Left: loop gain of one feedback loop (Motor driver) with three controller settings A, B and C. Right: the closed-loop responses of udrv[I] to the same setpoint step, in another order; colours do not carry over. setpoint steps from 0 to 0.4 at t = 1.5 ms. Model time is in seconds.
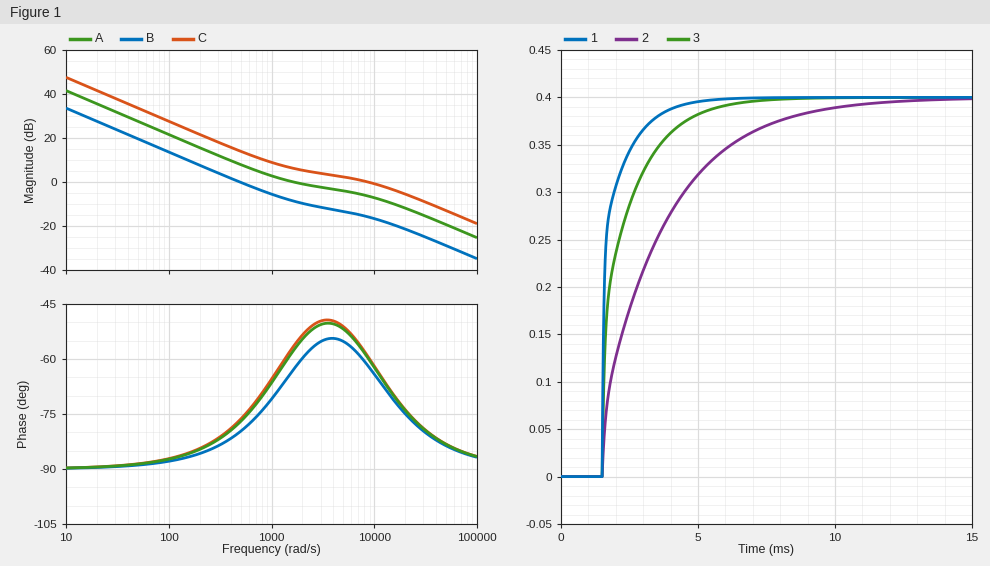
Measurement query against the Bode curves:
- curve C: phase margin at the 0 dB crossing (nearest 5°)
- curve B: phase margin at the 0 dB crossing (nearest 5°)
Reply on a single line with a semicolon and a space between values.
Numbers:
120°; 100°
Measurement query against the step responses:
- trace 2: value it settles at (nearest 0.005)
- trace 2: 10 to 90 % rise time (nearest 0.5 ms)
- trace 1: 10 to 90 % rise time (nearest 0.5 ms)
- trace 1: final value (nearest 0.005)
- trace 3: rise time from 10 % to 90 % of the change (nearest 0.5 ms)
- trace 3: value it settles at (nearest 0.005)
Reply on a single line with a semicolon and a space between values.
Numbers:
0.400; 5.0 ms; 1.5 ms; 0.400; 2.5 ms; 0.400
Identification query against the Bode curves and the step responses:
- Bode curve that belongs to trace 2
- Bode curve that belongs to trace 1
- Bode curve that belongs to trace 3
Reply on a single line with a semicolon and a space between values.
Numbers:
B; C; A
